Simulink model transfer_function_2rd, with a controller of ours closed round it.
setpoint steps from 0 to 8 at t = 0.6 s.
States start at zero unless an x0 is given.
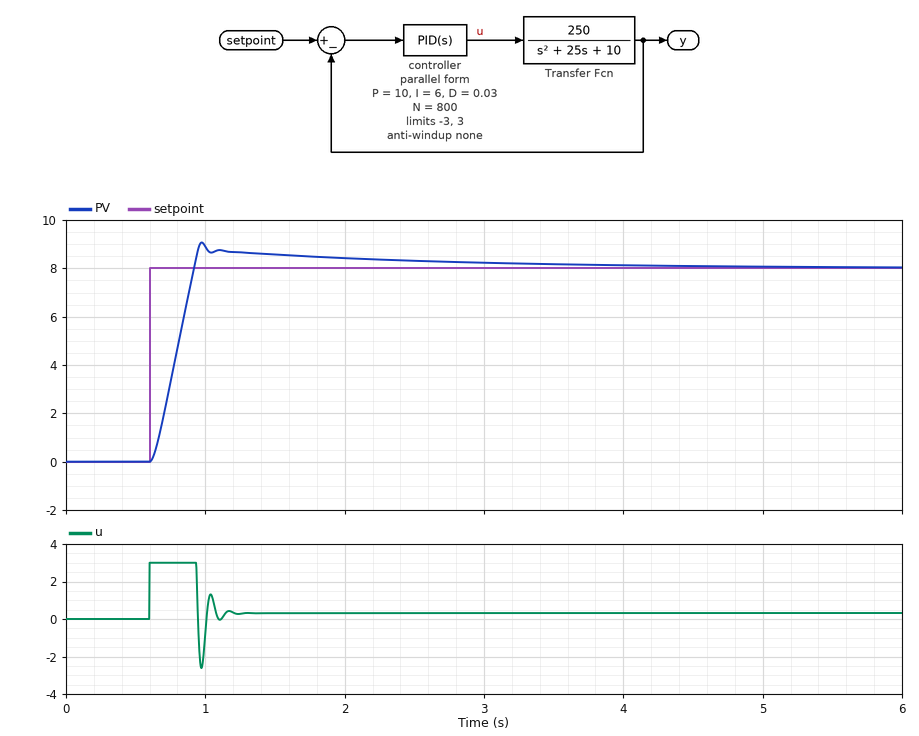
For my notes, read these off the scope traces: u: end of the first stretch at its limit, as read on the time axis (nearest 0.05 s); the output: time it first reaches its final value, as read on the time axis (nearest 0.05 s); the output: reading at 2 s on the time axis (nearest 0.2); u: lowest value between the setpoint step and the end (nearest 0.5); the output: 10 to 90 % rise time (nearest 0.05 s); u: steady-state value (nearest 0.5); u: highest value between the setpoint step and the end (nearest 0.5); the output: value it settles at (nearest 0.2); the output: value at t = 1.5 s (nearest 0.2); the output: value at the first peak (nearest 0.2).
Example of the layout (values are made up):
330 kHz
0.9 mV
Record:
0.95 s
0.90 s
8.4
-2.5
0.25 s
0.5
3.0
8.0
8.6
9.0
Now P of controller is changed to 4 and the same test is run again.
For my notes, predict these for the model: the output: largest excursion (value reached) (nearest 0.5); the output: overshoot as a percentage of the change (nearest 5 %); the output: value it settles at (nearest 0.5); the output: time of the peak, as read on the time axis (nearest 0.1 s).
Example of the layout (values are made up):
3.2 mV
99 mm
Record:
10.0
25 %
8.0
1.0 s
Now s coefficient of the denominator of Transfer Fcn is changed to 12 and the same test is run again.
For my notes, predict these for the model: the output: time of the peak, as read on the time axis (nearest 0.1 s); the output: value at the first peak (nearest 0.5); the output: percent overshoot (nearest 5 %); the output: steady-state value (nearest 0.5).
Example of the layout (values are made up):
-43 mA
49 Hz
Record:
0.9 s
9.5
20 %
8.0
